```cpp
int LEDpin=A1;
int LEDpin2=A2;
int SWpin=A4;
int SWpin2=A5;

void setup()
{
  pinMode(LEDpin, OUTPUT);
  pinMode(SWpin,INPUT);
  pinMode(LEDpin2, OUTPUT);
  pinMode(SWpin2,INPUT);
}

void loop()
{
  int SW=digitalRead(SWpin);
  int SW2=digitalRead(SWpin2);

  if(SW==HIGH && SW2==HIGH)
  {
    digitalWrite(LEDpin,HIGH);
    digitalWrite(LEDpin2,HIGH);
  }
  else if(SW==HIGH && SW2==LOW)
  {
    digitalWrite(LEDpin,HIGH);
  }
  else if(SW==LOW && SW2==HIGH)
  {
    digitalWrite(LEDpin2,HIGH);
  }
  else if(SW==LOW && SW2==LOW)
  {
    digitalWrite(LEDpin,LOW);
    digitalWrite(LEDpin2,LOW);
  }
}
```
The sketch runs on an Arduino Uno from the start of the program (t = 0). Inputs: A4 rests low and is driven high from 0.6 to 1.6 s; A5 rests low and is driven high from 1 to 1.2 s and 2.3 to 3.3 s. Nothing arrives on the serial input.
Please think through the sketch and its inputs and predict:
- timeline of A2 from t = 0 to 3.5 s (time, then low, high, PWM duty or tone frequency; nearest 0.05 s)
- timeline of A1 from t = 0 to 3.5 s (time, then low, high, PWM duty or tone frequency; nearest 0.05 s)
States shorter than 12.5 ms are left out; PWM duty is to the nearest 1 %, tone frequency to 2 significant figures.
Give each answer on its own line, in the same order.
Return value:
0 s low; 1 s high; 1.6 s low; 2.3 s high; 3.3 s low
0 s low; 0.6 s high; 1.6 s low
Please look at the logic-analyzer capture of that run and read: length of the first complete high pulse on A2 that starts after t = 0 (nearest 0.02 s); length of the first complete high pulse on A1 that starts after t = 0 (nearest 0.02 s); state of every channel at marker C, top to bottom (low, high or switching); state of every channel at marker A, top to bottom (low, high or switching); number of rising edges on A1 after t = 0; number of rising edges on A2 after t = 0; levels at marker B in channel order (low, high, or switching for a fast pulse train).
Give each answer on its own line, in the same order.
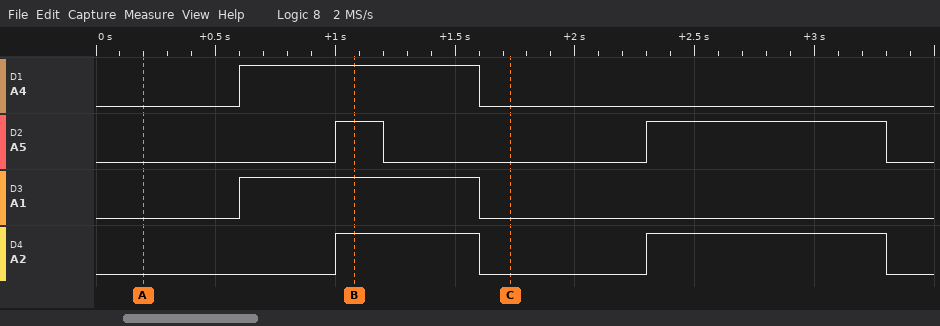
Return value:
0.60 s
1.00 s
A4 low, A5 low, A1 low, A2 low
A4 low, A5 low, A1 low, A2 low
1
2
A4 high, A5 high, A1 high, A2 high
